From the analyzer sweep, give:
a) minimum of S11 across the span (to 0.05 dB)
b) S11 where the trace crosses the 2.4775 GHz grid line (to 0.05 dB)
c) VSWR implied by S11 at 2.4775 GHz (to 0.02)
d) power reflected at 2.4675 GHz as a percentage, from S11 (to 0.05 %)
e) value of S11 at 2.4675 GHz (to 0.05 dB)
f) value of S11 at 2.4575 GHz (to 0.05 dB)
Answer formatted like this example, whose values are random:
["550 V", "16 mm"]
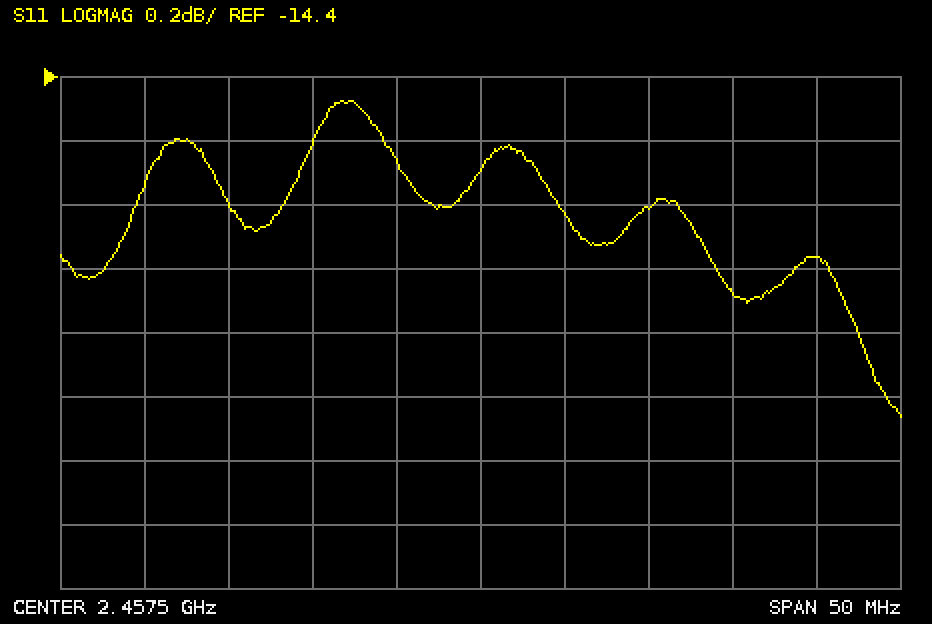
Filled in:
["-15.45 dB", "-14.95 dB", "1.44", "3.30 %", "-14.80 dB", "-14.70 dB"]
